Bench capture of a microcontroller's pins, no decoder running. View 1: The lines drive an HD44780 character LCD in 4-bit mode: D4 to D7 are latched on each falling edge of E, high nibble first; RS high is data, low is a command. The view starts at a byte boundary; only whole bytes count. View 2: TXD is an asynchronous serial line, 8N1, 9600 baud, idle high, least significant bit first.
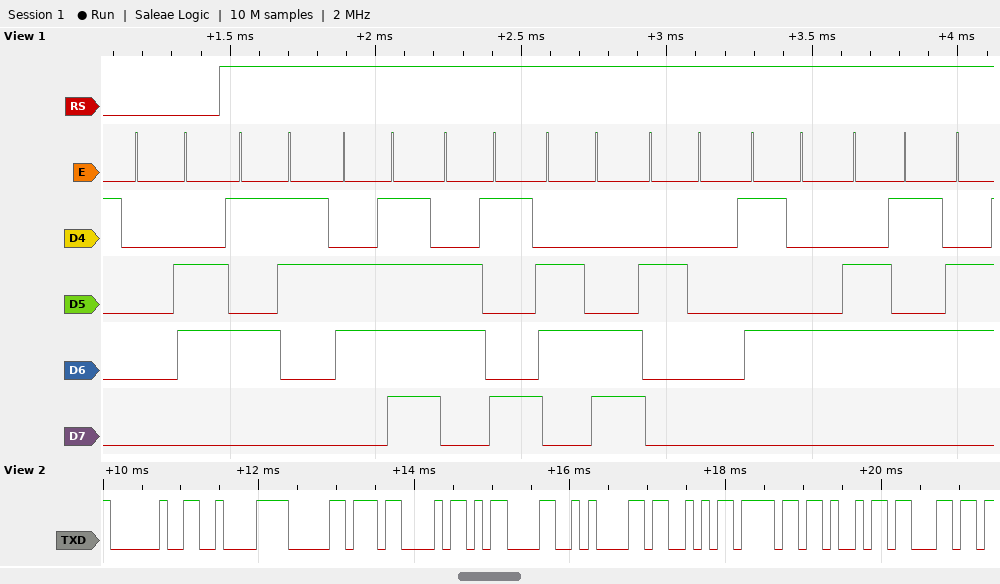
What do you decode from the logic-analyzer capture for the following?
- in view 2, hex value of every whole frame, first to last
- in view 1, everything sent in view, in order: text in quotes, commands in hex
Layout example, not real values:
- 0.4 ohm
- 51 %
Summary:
- 20 C2 B0 43 0D 0A 53 6F 69 6C
- 0x06 "Soil Te"
